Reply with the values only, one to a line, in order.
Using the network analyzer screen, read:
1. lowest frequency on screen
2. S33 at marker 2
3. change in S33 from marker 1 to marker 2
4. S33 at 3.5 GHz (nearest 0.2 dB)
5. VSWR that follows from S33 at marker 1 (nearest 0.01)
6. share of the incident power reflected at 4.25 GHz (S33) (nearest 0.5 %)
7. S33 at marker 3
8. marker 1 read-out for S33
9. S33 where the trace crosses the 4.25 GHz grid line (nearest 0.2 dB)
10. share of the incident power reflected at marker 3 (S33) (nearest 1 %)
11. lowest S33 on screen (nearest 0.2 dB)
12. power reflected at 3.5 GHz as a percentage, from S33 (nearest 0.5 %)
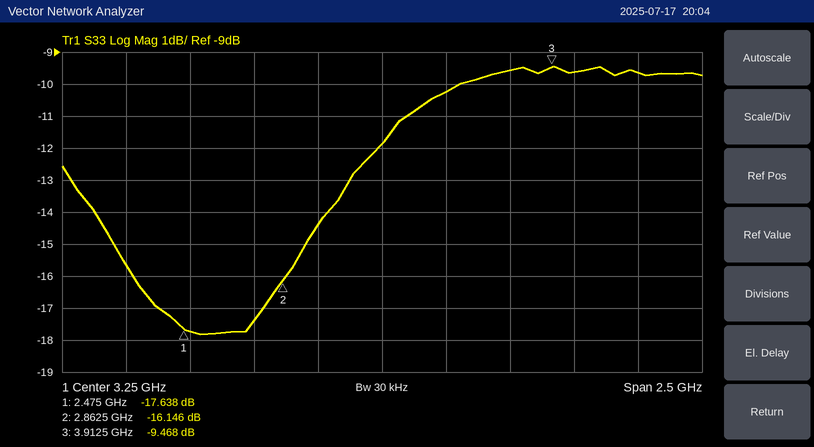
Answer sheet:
2 GHz
-16.146 dB
1.492 dB
-10.2 dB
1.30
11.0 %
-9.468 dB
-17.638 dB
-9.6 dB
11 %
-17.8 dB
9.5 %
